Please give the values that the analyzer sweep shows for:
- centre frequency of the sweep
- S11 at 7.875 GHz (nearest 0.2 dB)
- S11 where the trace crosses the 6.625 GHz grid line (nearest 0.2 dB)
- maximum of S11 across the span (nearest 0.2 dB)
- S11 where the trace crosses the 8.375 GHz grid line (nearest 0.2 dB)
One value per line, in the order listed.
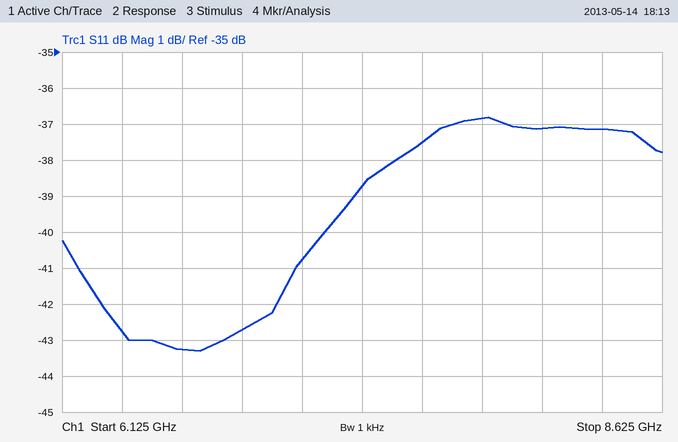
7.375 GHz
-36.8 dB
-43.2 dB
-36.8 dB
-37.2 dB
